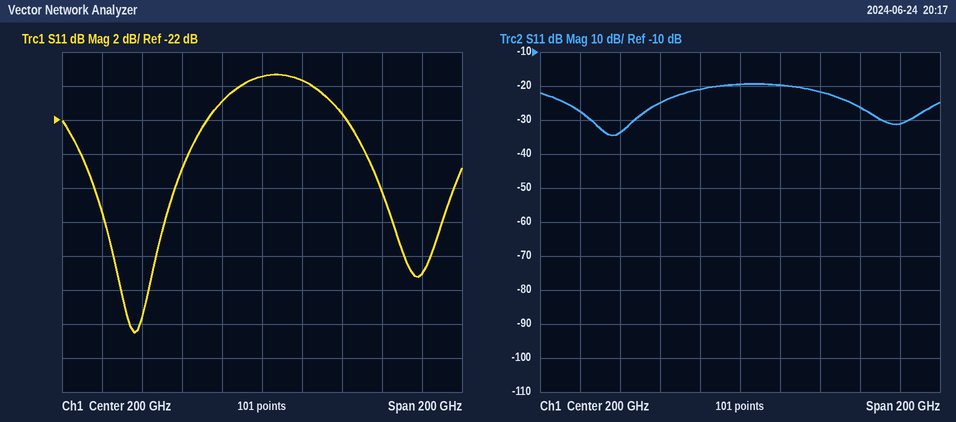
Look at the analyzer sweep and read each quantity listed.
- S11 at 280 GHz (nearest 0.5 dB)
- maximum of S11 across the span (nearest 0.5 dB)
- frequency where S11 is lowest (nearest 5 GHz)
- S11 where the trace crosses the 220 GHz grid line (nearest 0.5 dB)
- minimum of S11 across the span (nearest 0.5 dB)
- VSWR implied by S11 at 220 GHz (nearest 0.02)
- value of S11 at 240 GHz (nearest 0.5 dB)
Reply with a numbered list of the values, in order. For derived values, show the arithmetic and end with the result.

1. -31.0 dB
2. -19.5 dB
3. 135 GHz
4. -19.5 dB
5. -34.5 dB
6. |Γ| = 10^(-19.5/20) = 0.1059; VSWR = (1 + 0.1059)/(1 − 0.1059) ≈ 1.24
7. -21.5 dB
